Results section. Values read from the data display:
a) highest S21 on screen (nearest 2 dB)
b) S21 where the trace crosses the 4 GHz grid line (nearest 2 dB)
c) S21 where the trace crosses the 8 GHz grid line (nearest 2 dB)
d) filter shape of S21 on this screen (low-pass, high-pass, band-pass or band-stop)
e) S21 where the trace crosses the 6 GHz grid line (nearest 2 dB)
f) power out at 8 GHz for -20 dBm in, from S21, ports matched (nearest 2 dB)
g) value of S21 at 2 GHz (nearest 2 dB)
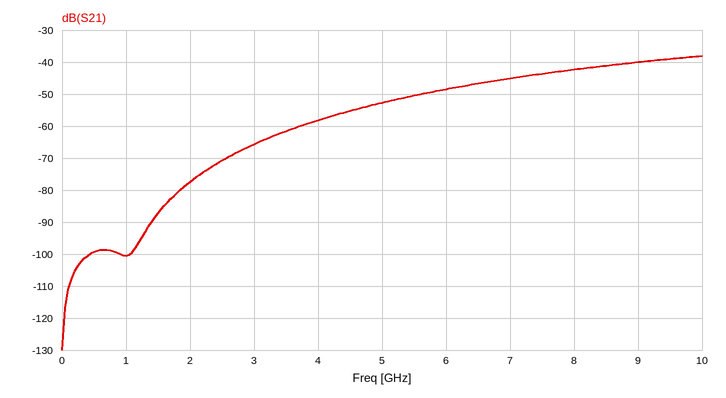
-38 dB
-58 dB
-42 dB
high-pass
-48 dB
-62 dBm
-78 dB
